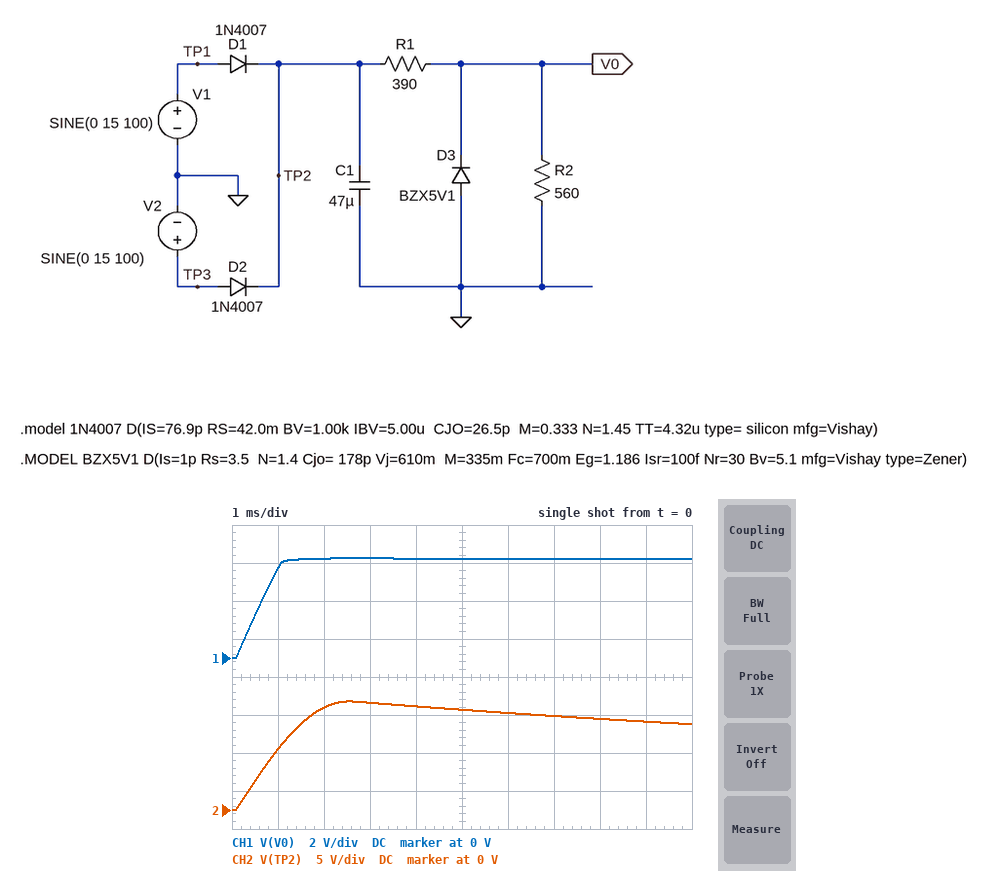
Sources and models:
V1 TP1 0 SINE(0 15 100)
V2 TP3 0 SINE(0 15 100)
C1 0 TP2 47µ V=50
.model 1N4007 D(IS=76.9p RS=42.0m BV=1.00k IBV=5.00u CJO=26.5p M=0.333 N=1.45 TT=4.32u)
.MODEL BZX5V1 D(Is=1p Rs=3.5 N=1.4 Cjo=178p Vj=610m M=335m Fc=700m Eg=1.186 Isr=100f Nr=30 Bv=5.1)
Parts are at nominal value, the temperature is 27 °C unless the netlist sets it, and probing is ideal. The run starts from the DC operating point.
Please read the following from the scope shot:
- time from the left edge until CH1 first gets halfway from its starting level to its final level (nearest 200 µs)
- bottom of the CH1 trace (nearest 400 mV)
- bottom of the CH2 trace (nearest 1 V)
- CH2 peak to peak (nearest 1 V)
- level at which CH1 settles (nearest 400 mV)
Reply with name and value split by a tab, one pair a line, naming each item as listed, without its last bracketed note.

time from the left edge until CH1 first gets halfway from its starting level to its final level	600 µs
bottom of the CH1 trace	0 V
bottom of the CH2 trace	0 V
CH2 peak to peak	14 V
level at which CH1 settles	5.2 V
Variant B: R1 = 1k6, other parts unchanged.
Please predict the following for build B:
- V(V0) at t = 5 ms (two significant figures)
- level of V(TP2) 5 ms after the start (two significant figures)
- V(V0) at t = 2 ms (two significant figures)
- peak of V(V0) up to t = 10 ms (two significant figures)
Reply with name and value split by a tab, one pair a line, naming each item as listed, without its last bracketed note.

V(V0) at t = 5 ms	3.6 V
level of V(TP2) 5 ms after the start	14 V
V(V0) at t = 2 ms	3.5 V
peak of V(V0) up to t = 10 ms	3.7 V
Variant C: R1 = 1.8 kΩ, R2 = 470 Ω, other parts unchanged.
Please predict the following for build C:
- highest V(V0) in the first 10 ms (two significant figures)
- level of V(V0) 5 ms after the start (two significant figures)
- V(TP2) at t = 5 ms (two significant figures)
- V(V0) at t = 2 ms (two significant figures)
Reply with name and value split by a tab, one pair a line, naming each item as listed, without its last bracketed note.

highest V(V0) in the first 10 ms	3.0 V
level of V(V0) 5 ms after the start	2.9 V
V(TP2) at t = 5 ms	14 V
V(V0) at t = 2 ms	2.8 V
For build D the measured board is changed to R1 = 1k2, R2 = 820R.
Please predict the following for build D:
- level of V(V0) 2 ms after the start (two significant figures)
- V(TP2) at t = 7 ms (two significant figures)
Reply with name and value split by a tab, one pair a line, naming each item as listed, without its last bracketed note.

level of V(V0) 2 ms after the start	5.1 V
V(TP2) at t = 7 ms	14 V
